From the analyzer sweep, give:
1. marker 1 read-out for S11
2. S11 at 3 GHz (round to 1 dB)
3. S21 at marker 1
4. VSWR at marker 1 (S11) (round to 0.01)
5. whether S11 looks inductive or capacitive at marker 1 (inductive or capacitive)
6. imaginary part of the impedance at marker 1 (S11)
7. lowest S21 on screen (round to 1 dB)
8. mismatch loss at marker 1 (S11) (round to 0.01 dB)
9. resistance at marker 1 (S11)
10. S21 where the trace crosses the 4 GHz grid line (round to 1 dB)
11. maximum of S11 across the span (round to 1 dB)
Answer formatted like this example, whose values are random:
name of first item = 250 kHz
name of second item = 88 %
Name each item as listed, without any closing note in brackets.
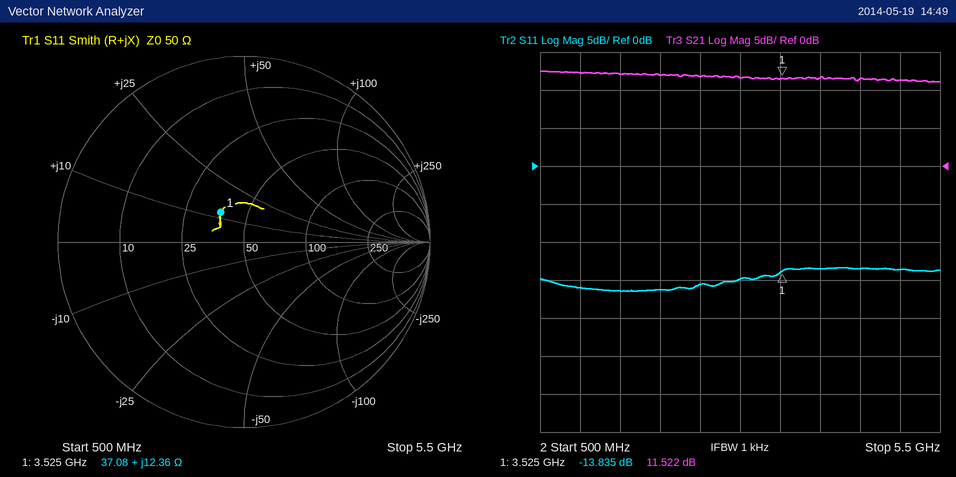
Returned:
marker 1 read-out for S11 = -13.835 dB
S11 at 3 GHz = -15 dB
S21 at marker 1 = 11.522 dB
VSWR at marker 1 (S11) = 1.51
whether S11 looks inductive or capacitive at marker 1 = inductive
imaginary part of the impedance at marker 1 = +12.36 Ω
lowest S21 on screen = 11 dB
mismatch loss at marker 1 (S11) = 0.18 dB
resistance at marker 1 = 37.08 Ω
S21 where the trace crosses the 4 GHz grid line = 12 dB
maximum of S11 across the span = -13 dB
